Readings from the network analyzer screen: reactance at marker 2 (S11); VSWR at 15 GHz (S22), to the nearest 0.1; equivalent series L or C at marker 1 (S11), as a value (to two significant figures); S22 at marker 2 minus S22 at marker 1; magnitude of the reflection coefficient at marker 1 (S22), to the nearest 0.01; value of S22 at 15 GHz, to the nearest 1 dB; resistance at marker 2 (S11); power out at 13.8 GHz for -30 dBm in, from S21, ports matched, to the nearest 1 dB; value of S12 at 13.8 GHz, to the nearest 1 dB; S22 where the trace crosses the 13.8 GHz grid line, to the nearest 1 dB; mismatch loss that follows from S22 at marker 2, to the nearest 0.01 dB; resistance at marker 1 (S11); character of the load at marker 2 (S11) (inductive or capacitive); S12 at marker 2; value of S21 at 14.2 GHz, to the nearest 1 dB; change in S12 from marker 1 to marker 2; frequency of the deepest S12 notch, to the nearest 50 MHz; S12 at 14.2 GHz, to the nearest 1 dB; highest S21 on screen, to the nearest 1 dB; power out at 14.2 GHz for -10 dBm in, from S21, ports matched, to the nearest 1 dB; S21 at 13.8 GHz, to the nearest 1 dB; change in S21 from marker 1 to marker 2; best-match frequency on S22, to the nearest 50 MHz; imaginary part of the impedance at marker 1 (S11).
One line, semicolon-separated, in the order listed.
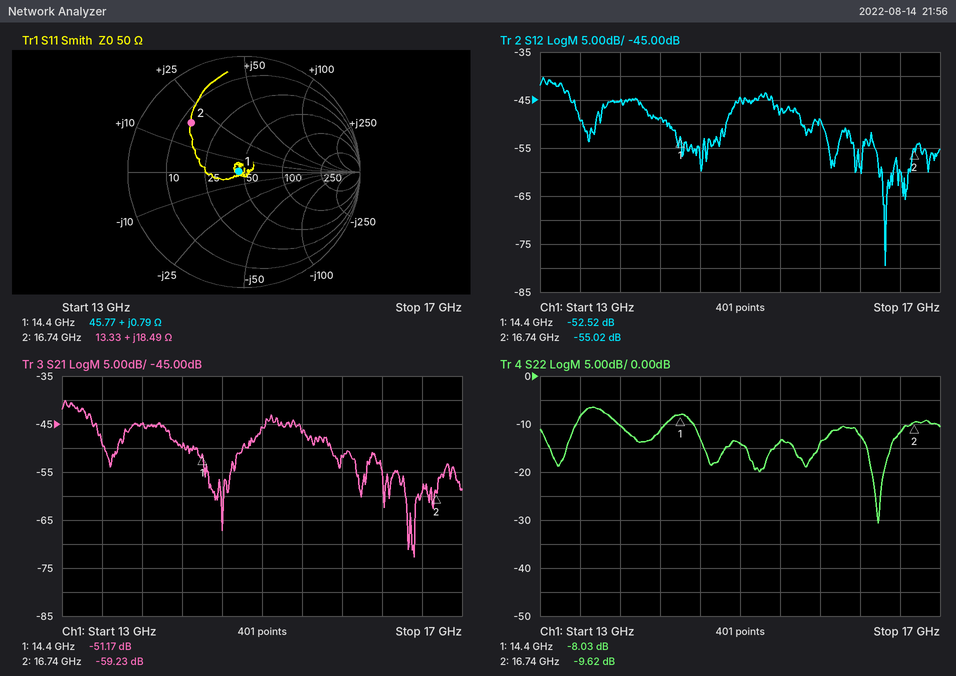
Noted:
+18.49 Ω; 1.5; 8.7 pH; -1.59 dB; 0.40; -14 dB; 13.33 Ω; -75 dBm; -45 dB; -10 dB; 0.50 dB; 45.77 Ω; inductive; -55.02 dB; -50 dB; -2.50 dB; 16.45 GHz; -49 dB; -40 dB; -60 dBm; -45 dB; -8.06 dB; 16.40 GHz; +0.79 Ω
